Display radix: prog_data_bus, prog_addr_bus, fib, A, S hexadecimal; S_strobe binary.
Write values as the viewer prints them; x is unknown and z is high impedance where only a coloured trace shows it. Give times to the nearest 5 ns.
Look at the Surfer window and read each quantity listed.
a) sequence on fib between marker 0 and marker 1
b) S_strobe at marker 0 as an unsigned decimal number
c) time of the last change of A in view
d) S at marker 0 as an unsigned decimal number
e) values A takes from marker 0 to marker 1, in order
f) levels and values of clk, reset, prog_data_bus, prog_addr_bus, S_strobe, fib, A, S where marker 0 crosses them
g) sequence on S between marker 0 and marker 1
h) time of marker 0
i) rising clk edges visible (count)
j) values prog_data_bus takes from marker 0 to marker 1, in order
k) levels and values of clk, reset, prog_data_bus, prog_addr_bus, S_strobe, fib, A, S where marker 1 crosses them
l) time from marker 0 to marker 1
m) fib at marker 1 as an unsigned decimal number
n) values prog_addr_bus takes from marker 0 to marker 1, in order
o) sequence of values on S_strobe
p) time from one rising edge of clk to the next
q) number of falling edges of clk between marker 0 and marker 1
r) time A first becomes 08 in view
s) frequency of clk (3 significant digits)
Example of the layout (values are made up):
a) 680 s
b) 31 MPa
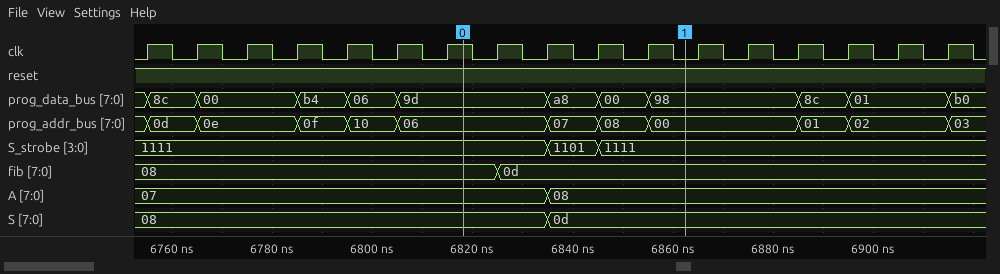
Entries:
a) 08, 0d
b) 15
c) 6835 ns
d) 8
e) 07, 08
f) clk=1, reset=1, prog_data_bus=9d, prog_addr_bus=06, S_strobe=1111, fib=08, A=07, S=08
g) 08, 0d
h) 6820 ns
i) 17
j) 9d, a8, 00, 98
k) clk=0, reset=1, prog_data_bus=98, prog_addr_bus=00, S_strobe=1111, fib=0d, A=08, S=0d
l) 45 ns
m) 13
n) 06, 07, 08, 00
o) 1111, 1101, 1111
p) 10 ns
q) 5
r) 6835 ns
s) 100 MHz
